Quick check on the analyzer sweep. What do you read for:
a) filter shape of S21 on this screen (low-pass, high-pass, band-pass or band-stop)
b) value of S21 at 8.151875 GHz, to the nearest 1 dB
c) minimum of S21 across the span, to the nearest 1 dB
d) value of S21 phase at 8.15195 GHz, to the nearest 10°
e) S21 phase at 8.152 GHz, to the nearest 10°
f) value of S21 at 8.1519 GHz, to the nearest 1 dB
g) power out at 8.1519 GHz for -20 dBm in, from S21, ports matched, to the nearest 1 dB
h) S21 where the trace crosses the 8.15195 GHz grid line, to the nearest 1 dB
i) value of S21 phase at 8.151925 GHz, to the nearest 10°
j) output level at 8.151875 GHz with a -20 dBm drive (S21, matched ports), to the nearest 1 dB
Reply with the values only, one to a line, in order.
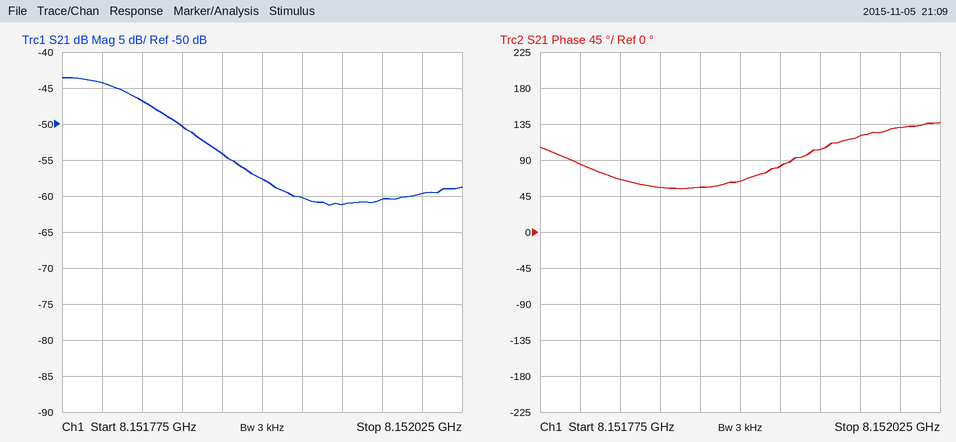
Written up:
low-pass
-54 dB
-61 dB
100°
130°
-58 dB
-78 dBm
-61 dB
80°
-74 dBm
